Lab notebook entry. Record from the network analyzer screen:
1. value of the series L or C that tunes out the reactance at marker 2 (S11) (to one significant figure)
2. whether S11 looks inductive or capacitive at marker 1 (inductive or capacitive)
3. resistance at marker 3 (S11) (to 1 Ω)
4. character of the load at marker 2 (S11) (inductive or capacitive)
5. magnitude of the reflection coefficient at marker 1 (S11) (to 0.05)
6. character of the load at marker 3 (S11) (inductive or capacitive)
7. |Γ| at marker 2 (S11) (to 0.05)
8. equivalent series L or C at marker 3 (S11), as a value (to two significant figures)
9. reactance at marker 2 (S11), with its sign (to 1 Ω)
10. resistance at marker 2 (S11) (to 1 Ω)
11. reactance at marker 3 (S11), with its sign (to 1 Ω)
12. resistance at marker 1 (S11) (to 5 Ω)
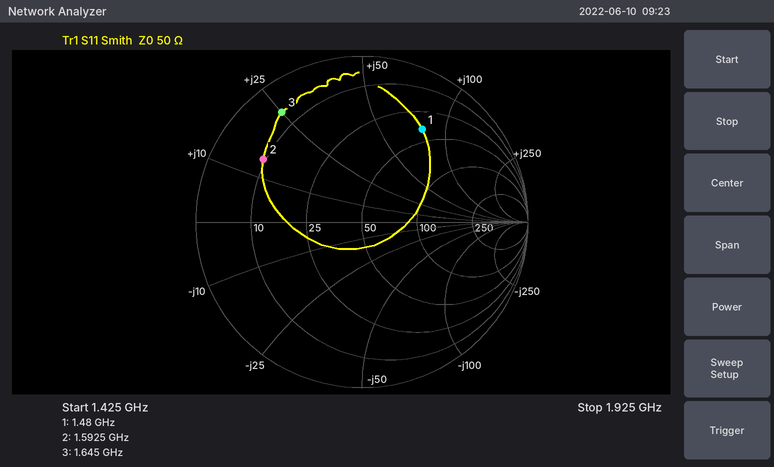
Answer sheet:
7 pF
inductive
6 Ω
inductive
0.65
inductive
0.70
2.4 nH
+14 Ω
9 Ω
+25 Ω
40 Ω
